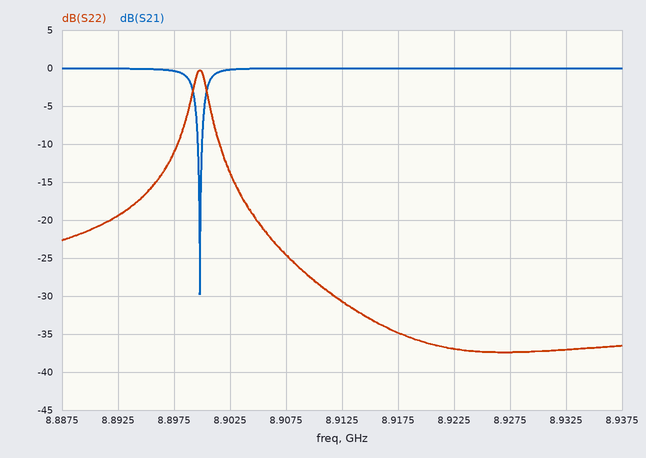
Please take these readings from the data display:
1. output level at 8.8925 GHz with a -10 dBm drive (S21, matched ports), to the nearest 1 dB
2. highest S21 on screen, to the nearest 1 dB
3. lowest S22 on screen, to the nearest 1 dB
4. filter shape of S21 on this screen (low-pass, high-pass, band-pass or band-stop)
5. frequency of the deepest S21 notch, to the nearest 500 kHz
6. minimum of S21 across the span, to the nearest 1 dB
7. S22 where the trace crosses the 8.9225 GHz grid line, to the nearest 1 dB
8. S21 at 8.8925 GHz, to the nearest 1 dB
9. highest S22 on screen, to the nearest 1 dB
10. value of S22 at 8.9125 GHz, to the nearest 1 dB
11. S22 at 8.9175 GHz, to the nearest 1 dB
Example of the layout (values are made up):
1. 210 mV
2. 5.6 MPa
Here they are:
1. -10 dBm
2. 0 dB
3. -37 dB
4. band-stop
5. 8.9000 GHz
6. -30 dB
7. -37 dB
8. 0 dB
9. 0 dB
10. -31 dB
11. -35 dB
